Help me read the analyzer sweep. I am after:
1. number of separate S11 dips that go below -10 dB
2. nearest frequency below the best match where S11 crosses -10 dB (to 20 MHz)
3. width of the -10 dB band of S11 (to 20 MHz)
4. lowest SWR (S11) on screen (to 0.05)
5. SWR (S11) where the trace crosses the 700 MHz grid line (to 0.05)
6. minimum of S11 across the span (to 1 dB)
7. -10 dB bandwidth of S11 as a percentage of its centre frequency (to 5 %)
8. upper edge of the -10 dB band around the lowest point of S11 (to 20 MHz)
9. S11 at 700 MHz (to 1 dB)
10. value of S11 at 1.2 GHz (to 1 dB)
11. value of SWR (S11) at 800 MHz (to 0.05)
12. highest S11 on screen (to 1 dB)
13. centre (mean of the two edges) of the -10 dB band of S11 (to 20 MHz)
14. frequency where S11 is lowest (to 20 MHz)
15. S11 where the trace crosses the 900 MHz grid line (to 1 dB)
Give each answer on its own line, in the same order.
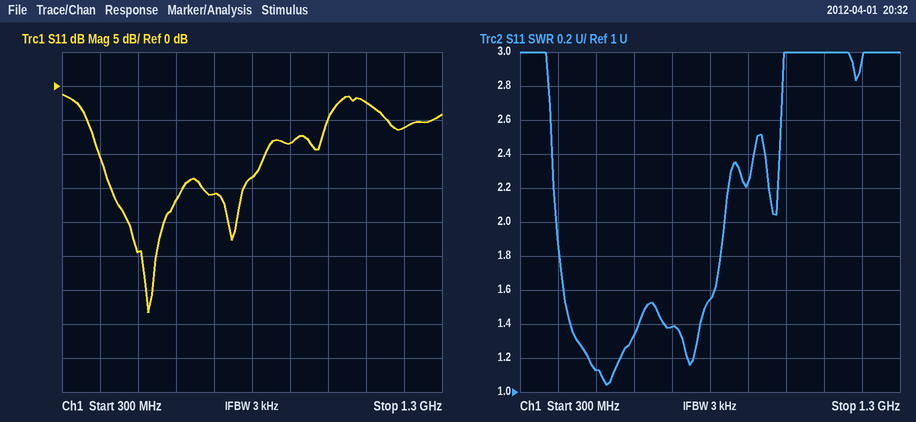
2
400 MHz
440 MHz
1.05
1.40
-33 dB
70 %
840 MHz
-16 dB
-6 dB
1.55
-1 dB
620 MHz
520 MHz
-8 dB
